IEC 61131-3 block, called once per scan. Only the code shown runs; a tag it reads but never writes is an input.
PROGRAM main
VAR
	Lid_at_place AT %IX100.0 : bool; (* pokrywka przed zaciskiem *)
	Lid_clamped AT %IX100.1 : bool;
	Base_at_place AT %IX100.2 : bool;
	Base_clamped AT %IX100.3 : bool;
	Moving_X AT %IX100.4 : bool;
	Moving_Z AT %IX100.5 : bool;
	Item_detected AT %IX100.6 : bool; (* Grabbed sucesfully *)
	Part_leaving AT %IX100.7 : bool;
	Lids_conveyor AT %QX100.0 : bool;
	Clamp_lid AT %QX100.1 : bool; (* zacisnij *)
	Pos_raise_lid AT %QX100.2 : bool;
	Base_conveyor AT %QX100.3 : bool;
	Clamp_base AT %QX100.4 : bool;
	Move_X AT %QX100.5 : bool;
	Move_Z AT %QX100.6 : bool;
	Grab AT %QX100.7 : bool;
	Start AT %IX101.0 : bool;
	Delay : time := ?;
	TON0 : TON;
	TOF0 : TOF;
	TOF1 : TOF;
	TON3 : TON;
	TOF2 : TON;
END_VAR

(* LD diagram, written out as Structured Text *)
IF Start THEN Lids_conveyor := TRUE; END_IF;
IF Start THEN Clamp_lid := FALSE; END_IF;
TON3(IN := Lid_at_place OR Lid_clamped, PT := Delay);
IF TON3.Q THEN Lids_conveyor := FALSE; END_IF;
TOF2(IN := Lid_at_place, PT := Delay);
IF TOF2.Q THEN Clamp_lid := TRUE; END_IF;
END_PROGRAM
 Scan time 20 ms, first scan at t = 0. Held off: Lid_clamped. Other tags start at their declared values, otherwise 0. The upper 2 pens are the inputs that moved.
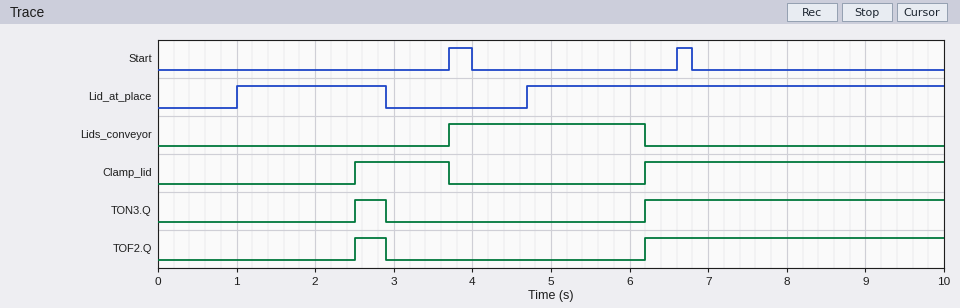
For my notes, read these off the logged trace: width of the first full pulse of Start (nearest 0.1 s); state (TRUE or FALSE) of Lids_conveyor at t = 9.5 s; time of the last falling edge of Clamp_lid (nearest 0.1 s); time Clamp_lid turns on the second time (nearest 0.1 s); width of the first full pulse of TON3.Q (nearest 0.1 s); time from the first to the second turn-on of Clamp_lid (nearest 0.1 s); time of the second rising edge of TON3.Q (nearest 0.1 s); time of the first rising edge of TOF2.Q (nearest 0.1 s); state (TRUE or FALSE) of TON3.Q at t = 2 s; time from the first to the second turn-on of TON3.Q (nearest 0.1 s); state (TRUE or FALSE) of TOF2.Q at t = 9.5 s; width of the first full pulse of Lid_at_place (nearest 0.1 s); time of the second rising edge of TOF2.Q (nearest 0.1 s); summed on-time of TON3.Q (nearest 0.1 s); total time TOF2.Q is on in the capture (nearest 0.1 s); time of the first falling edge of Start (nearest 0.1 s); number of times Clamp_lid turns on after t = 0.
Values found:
0.3 s
FALSE
3.7 s
6.2 s
0.4 s
3.7 s
6.2 s
2.5 s
FALSE
3.7 s
TRUE
1.9 s
6.2 s
4.2 s
4.2 s
4.0 s
2
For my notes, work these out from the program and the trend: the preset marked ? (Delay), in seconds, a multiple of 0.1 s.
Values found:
1.5 s
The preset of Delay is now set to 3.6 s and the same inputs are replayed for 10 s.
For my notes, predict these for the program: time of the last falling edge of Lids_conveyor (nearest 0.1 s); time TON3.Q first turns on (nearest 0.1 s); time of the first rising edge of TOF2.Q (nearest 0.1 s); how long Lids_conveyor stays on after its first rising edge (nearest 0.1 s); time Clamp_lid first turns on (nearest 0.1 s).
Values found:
8.3 s
8.3 s
8.3 s
4.6 s
8.3 s
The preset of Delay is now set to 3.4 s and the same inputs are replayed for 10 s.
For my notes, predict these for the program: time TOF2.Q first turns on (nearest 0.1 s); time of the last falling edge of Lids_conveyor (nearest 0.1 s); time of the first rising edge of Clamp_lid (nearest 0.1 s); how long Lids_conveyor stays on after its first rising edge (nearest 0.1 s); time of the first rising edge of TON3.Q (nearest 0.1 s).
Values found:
8.1 s
8.1 s
8.1 s
4.4 s
8.1 s
